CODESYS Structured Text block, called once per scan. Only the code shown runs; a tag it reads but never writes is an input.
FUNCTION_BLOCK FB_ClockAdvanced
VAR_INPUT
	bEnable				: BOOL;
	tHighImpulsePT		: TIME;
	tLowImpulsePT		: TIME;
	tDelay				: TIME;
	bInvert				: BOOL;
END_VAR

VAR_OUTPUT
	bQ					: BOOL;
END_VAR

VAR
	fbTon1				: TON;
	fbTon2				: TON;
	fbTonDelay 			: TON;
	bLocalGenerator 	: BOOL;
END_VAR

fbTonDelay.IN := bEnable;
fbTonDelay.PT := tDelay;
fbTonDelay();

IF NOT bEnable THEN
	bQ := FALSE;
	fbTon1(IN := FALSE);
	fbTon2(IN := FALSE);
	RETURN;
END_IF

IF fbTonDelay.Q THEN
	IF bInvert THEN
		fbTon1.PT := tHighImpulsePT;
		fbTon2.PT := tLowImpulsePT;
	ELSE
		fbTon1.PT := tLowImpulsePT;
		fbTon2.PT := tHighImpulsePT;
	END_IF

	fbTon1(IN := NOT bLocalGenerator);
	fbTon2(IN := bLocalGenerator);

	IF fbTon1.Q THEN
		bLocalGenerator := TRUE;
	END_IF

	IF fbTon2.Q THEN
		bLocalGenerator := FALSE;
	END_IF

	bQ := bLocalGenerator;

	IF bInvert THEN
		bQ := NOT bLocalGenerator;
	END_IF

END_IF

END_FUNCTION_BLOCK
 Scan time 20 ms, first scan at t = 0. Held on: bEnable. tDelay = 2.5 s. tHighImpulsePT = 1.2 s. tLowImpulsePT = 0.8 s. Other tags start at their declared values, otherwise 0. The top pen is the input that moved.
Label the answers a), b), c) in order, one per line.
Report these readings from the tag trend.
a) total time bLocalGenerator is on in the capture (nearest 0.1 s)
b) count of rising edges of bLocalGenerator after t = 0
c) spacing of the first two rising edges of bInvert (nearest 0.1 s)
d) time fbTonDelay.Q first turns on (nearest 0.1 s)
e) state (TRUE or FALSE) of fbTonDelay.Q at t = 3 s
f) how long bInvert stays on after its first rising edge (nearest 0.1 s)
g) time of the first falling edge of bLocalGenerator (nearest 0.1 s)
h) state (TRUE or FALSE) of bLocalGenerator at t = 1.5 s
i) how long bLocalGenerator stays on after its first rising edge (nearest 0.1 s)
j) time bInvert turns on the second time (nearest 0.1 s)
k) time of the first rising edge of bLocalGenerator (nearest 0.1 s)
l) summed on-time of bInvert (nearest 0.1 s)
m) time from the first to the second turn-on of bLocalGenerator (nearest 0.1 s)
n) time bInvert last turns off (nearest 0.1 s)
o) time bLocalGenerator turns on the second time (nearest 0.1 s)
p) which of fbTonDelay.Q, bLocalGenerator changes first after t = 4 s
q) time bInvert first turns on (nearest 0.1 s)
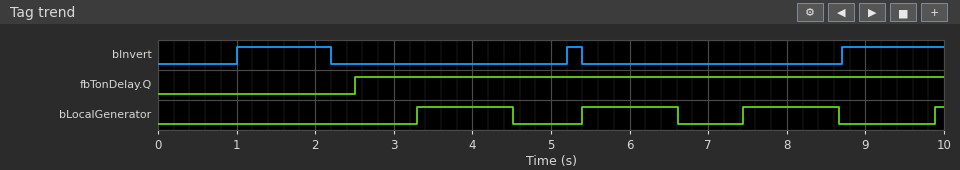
a) 3.8 s
b) 4
c) 4.2 s
d) 2.5 s
e) TRUE
f) 1.2 s
g) 4.5 s
h) FALSE
i) 1.2 s
j) 5.2 s
k) 3.3 s
l) 2.7 s
m) 2.1 s
n) 5.4 s
o) 5.4 s
p) bLocalGenerator
q) 1.0 s
